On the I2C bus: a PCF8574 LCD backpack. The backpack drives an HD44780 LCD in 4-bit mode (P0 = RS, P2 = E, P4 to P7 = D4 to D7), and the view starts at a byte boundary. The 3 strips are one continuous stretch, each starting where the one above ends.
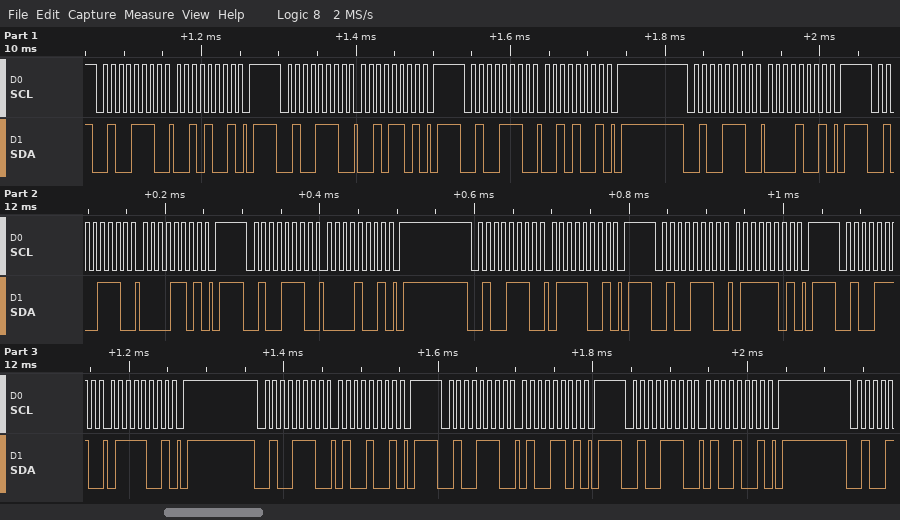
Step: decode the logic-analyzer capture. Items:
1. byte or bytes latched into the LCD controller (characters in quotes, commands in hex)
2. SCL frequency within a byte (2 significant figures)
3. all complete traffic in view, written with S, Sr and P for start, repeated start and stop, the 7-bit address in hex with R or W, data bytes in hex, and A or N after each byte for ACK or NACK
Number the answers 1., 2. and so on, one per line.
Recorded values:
1. ' ' 't'
2. 100 kHz
3. S 27W A 29 A P S 27W A 2D A P S 27W A 29 A P S 27W A 09 A P S 27W A 0D A P S 27W A 09 A P S 27W A 79 A P S 27W A 7D A P S 27W A 79 A P S 27W A 49 A P S 27W A 4D A P S 27W A 49 A P
